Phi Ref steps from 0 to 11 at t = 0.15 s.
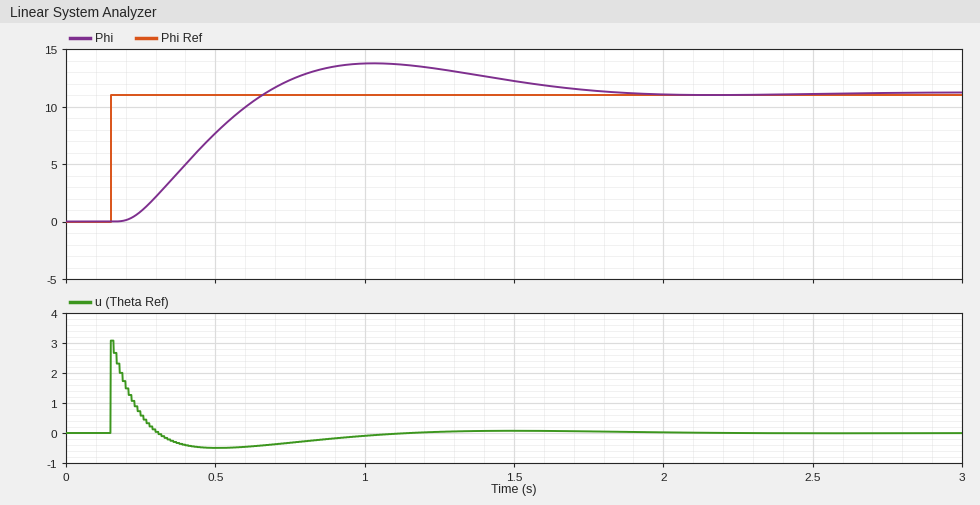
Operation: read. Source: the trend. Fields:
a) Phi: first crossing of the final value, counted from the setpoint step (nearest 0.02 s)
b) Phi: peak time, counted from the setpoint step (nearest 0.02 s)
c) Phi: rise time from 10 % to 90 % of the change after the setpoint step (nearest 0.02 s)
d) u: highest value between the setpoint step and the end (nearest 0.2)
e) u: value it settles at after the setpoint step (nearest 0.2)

0.52 s
0.88 s
0.34 s
3.0
0.0
